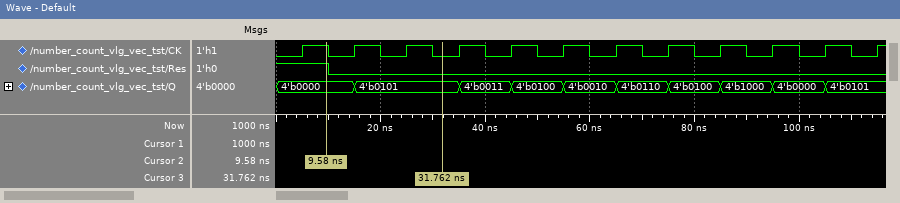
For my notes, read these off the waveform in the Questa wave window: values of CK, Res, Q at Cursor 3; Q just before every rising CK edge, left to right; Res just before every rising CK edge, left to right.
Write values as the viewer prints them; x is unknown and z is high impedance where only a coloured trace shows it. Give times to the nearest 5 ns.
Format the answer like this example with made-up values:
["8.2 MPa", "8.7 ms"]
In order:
["CK=0, Res=0, Q=4'b0101", "4'b0000, 4'b0000, 4'b0101, 4'b0101, 4'b0011, 4'b0100, 4'b0010, 4'b0110, 4'b0100, 4'b1000, 4'b0000, 4'b0101", "1 0 0 0 0 0 0 0 0 0 0 0"]
